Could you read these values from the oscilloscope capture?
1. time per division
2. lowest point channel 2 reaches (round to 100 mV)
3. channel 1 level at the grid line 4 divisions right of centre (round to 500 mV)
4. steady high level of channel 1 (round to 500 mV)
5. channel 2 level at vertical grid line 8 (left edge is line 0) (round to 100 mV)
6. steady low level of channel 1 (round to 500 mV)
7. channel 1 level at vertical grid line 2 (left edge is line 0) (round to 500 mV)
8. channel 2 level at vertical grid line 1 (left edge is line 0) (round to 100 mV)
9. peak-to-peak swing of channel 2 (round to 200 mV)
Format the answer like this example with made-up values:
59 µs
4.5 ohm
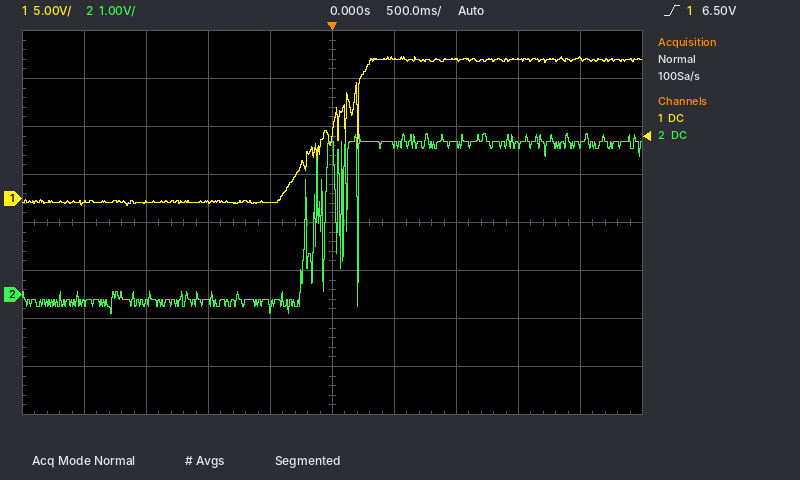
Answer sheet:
500 ms
-400 mV
14.5 V
14.5 V
3.1 V
-500 mV
-500 mV
-200 mV
3.8 V
